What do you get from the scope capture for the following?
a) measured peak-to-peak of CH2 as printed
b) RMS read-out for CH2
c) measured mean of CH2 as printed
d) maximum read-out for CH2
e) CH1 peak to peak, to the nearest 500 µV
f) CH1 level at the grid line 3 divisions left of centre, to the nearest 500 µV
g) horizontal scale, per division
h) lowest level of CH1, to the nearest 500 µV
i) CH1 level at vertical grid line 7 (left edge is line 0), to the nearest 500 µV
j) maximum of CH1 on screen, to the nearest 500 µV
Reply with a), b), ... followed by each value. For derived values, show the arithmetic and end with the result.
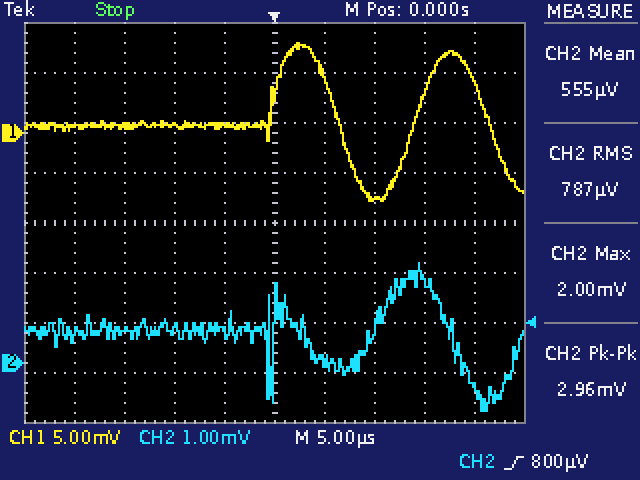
a) 2.96 mV
b) 787 µV
c) 555 µV
d) 2.00 mV
e) 9.0 mV − (-7.0 mV) = 16.0 mV
f) 500 µV
g) 5 µs
h) -7.0 mV
i) -6.5 mV
j) 9.0 mV
